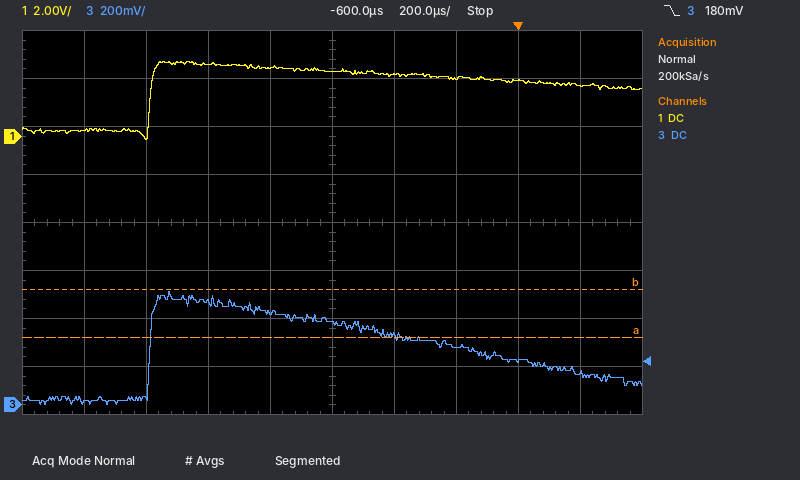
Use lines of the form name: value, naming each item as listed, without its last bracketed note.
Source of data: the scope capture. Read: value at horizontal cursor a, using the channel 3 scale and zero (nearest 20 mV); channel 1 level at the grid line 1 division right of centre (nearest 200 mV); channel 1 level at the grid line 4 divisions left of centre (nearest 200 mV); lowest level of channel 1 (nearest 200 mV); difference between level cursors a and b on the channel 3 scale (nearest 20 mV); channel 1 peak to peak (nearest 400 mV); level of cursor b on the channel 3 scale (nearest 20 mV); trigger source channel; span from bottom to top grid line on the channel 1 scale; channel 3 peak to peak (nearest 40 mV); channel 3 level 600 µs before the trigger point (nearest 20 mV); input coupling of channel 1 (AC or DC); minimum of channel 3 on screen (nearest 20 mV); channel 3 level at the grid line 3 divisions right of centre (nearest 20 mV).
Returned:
value at horizontal cursor a, using the channel 3 scale and zero: 280 mV
channel 1 level at the grid line 1 division right of centre: 2.6 V
channel 1 level at the grid line 4 divisions left of centre: 200 mV
lowest level of channel 1: -200 mV
difference between level cursors a and b on the channel 3 scale: 200 mV
channel 1 peak to peak: 3.2 V
level of cursor b on the channel 3 scale: 480 mV
trigger source channel: channel 3
span from bottom to top grid line on the channel 1 scale: 16 V
channel 3 peak to peak: 480 mV
channel 3 level 600 µs before the trigger point: 340 mV
input coupling of channel 1: DC
minimum of channel 3 on screen: 0 mV
channel 3 level at the grid line 3 divisions right of centre: 180 mV
